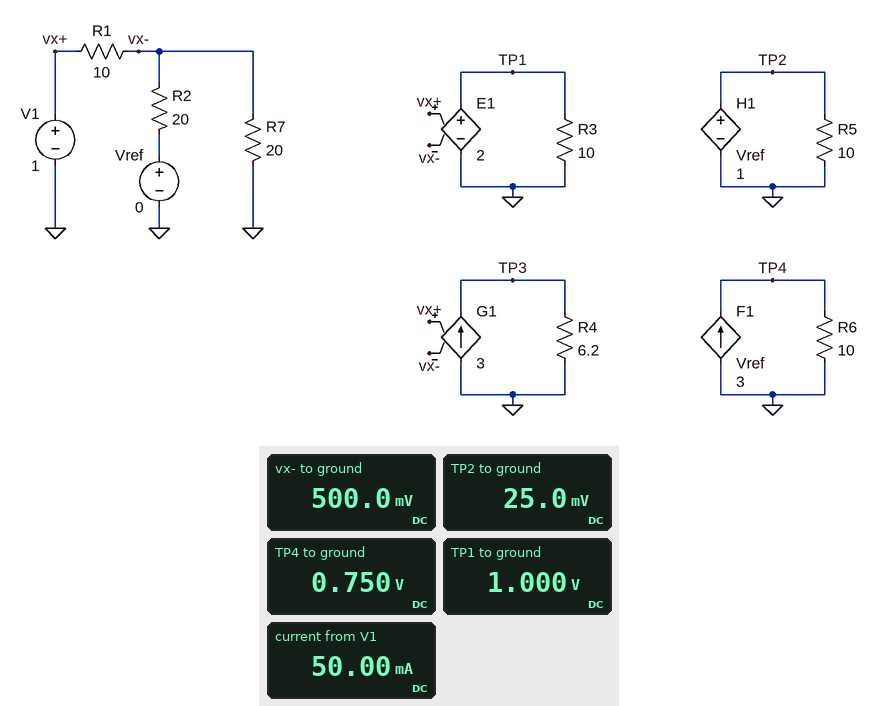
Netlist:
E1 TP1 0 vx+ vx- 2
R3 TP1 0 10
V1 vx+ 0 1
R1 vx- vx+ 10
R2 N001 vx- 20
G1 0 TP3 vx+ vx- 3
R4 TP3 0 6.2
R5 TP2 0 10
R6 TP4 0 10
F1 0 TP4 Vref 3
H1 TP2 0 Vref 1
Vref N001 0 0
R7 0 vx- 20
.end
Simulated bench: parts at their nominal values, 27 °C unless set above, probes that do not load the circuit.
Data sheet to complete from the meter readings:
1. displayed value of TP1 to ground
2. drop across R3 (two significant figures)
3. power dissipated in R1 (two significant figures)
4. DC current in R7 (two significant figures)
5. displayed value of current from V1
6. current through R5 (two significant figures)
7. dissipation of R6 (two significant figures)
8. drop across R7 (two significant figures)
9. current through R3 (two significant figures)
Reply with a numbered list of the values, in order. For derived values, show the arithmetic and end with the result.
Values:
1. 1.000 V
2. 1 V = 1.0 V
3. (1 V - 500 mV)^2 / 10 Ω = 25 mW
4. (500 mV) / 20 Ω = 25 mA
5. 50.00 mA
6. (25 mV) / 10 Ω = 2.5 mA
7. (750 mV)^2 / 10 Ω = 56 mW
8. 500 mV = 500 mV
9. (1 V) / 10 Ω = 100 mA
